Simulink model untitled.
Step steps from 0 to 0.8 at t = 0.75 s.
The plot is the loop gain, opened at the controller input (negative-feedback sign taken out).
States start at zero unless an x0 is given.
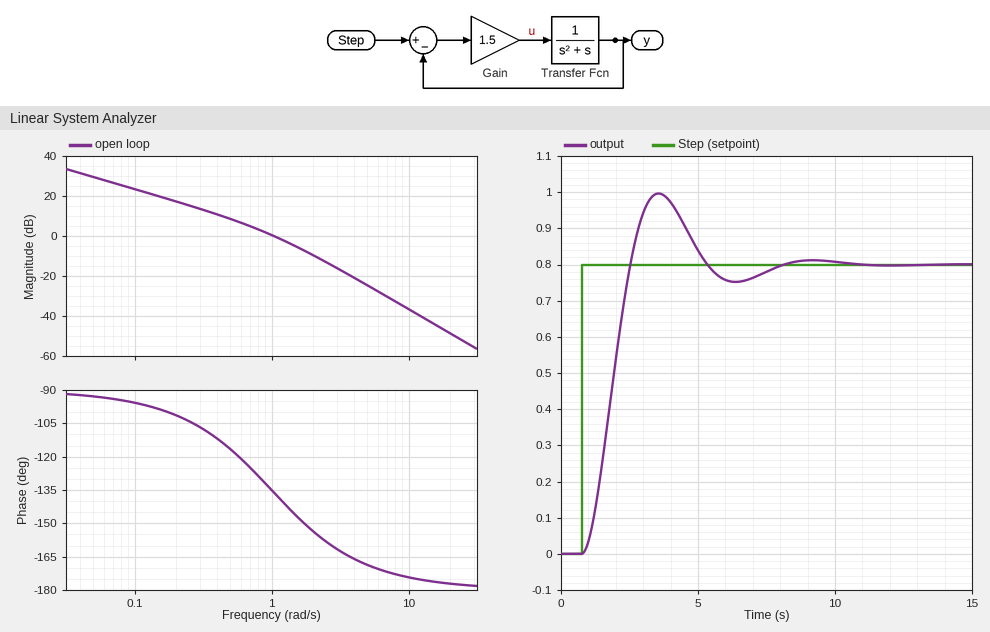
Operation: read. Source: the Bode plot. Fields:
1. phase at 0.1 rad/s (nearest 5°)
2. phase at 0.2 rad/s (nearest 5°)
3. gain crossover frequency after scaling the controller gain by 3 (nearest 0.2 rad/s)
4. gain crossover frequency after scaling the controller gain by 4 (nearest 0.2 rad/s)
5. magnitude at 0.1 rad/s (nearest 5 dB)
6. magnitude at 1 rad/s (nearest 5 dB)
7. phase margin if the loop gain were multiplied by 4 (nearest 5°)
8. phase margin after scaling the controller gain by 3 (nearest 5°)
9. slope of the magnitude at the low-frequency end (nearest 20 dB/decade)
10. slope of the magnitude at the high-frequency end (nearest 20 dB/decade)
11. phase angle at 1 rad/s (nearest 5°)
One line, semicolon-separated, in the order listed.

-95°; -100°; 2.0 rad/s; 2.4 rad/s; 25 dB; 0 dB; 25°; 25°; -20 dB/decade; -40 dB/decade; -135°
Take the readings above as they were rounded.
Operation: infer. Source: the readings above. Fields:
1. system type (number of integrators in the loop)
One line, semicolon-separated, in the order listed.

1
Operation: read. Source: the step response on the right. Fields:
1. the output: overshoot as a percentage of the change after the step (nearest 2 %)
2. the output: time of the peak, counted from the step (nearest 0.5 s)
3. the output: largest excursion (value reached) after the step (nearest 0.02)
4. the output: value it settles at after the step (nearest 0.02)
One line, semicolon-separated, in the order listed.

24 %; 3.0 s; 1.00; 0.80
